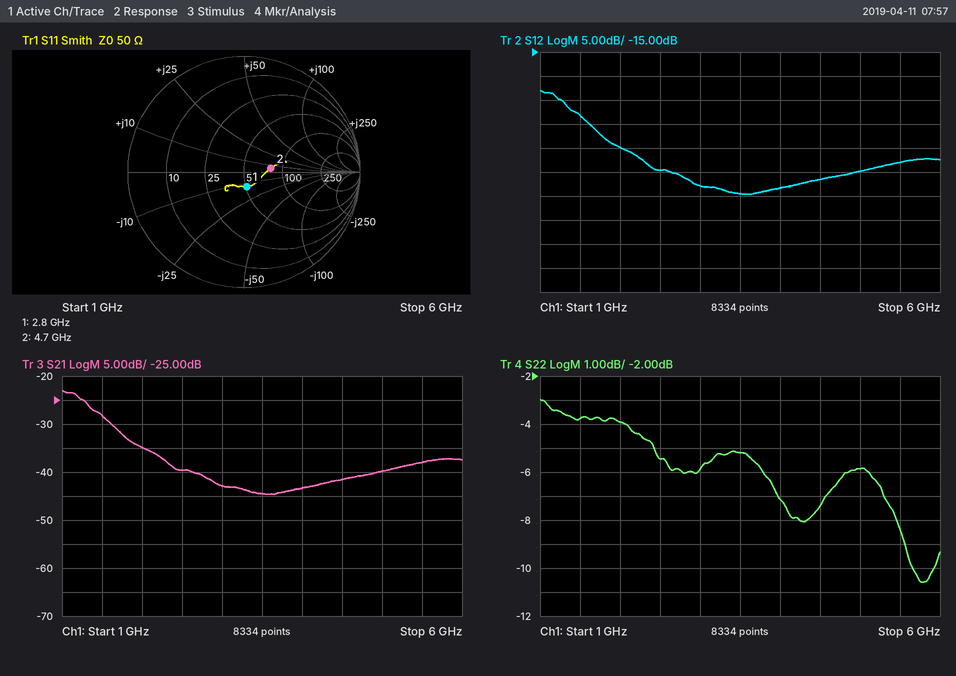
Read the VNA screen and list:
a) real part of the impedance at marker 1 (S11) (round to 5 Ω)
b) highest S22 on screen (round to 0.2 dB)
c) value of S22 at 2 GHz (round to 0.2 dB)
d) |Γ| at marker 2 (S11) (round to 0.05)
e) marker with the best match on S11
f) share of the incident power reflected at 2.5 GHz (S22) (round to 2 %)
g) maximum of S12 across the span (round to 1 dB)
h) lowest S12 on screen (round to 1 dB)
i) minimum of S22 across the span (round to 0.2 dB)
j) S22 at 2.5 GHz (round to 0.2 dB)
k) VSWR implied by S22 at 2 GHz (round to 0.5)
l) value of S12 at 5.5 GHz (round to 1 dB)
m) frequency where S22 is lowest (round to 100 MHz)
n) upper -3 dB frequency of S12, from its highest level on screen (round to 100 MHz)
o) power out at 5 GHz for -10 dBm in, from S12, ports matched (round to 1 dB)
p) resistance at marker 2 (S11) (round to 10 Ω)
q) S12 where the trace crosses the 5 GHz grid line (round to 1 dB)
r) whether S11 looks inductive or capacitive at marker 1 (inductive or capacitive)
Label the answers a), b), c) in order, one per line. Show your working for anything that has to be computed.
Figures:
a) 50 Ω
b) -3.0 dB
c) -4.0 dB
d) 0.25
e) marker 1
f) 10^(-5.4/10) ≈ 28.8 %, so 28 % to the nearest 2 %
g) -23 dB
h) -45 dB
i) -10.6 dB
j) -5.4 dB
k) |Γ| = 10^(-4/20) = 0.6310; VSWR = (1 + 0.6310)/(1 − 0.6310) ≈ 4.42, so 4.5 to the nearest 0.5
l) -38 dB
m) 5.8 GHz
n) 1.3 GHz
o) -10 dBm + (-40 dB) = -50 dBm
p) 80 Ω
q) -40 dB
r) capacitive
